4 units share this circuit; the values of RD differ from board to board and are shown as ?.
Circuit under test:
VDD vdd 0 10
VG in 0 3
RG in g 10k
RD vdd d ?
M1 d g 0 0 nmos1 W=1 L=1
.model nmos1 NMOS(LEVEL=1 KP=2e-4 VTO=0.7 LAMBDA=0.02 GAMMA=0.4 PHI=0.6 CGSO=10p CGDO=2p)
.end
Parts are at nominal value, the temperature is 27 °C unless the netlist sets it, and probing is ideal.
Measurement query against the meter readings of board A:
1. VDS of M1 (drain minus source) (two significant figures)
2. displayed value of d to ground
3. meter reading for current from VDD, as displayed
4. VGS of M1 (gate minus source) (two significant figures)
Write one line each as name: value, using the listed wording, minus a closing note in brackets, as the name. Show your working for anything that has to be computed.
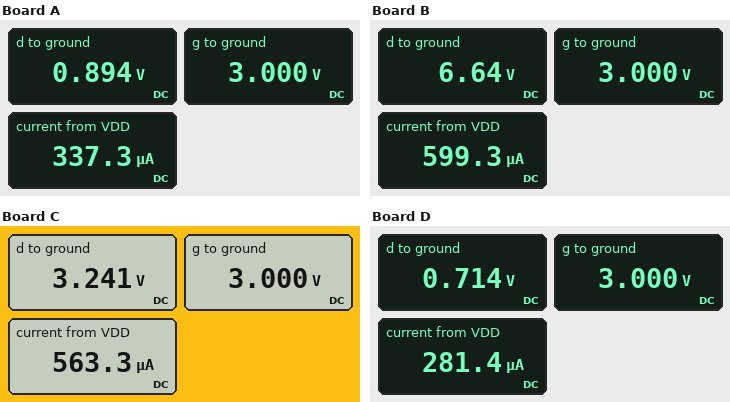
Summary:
VDS of M1 (drain minus source): 894 mV = 890 mV
displayed value of d to ground: 0.894 V
meter reading for current from VDD, as displayed: 337.3 µA
VGS of M1 (gate minus source): 3 V = 3.0 V
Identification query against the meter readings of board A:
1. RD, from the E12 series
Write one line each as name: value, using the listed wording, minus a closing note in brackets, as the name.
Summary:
RD, from the E12 series: 27 kΩ
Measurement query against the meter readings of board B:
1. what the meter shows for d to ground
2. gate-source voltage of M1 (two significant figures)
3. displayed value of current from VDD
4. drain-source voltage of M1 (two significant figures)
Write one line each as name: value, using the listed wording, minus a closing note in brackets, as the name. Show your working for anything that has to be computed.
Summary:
what the meter shows for d to ground: 6.64 V
gate-source voltage of M1: 3 V = 3.0 V
displayed value of current from VDD: 599.3 µA
drain-source voltage of M1: 6.64 V = 6.6 V
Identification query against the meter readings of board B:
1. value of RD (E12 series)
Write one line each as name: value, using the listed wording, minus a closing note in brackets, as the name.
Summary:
value of RD: 5.6 kΩ
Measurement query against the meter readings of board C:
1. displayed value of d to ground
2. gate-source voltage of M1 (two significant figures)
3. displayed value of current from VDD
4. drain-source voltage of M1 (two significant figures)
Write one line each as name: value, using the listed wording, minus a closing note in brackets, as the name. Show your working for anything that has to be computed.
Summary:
displayed value of d to ground: 3.241 V
gate-source voltage of M1: 3 V = 3.0 V
displayed value of current from VDD: 563.3 µA
drain-source voltage of M1: 3.241 V = 3.2 V
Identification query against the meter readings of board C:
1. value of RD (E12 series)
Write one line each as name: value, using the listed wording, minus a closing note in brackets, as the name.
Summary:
value of RD: 12 kΩ
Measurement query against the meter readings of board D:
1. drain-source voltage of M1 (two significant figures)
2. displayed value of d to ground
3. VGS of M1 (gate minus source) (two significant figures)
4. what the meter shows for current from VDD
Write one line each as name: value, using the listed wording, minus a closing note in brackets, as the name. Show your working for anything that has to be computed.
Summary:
drain-source voltage of M1: 714 mV = 710 mV
displayed value of d to ground: 0.714 V
VGS of M1 (gate minus source): 3 V = 3.0 V
what the meter shows for current from VDD: 281.4 µA
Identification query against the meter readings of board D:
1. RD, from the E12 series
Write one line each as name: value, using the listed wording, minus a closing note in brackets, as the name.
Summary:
RD, from the E12 series: 33 kΩ
